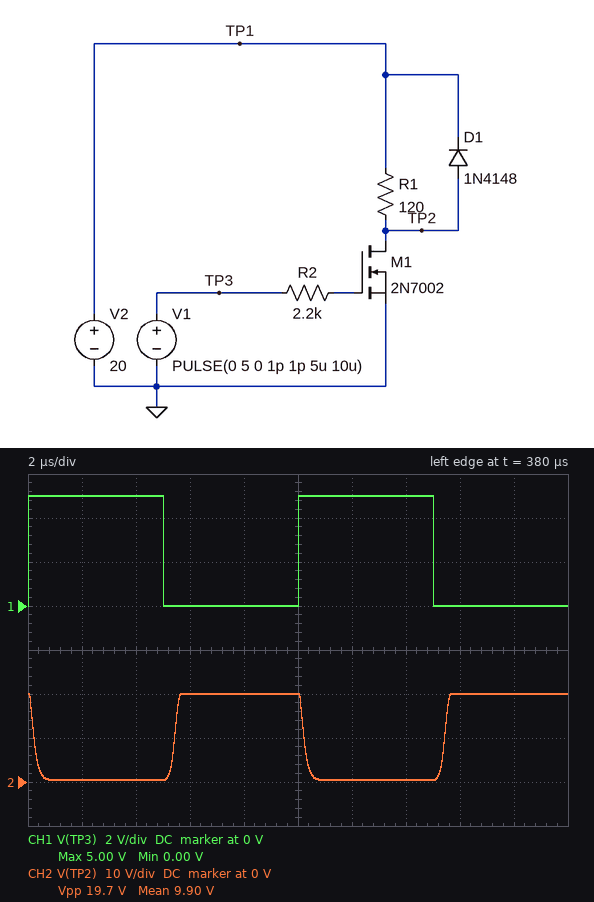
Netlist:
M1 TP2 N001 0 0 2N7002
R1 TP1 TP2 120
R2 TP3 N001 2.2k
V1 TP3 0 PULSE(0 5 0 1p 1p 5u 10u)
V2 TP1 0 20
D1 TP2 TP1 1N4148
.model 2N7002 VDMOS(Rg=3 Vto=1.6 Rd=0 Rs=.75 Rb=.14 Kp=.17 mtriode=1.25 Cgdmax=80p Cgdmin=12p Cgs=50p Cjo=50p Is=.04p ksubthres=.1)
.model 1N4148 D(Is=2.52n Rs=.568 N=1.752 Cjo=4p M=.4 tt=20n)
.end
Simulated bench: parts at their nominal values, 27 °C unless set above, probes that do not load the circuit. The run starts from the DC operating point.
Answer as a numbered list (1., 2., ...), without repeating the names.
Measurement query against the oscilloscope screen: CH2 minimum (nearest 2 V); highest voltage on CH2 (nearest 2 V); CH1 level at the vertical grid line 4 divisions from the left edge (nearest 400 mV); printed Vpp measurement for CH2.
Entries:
1. 0 V
2. 20 V
3. 0 V
4. 19.7 V
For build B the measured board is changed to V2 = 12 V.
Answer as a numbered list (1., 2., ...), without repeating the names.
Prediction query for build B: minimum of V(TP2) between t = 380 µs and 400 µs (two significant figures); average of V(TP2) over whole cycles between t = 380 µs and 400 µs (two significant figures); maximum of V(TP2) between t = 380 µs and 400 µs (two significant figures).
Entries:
1. 210 mV
2. 5.9 V
3. 12 V
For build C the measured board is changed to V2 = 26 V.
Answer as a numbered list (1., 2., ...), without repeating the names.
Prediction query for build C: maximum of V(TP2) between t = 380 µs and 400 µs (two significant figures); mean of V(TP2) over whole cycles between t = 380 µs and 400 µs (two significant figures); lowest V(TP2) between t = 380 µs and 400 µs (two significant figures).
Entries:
1. 26 V
2. 13 V
3. 490 mV
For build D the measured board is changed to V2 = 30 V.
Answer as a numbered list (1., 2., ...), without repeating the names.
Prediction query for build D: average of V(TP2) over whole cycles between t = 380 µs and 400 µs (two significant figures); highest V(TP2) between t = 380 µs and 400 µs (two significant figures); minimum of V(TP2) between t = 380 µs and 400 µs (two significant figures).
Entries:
1. 15 V
2. 30 V
3. 570 mV
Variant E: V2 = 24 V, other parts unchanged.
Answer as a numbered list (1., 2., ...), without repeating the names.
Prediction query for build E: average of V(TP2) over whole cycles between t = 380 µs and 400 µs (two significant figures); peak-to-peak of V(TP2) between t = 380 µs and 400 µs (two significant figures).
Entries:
1. 12 V
2. 24 V
